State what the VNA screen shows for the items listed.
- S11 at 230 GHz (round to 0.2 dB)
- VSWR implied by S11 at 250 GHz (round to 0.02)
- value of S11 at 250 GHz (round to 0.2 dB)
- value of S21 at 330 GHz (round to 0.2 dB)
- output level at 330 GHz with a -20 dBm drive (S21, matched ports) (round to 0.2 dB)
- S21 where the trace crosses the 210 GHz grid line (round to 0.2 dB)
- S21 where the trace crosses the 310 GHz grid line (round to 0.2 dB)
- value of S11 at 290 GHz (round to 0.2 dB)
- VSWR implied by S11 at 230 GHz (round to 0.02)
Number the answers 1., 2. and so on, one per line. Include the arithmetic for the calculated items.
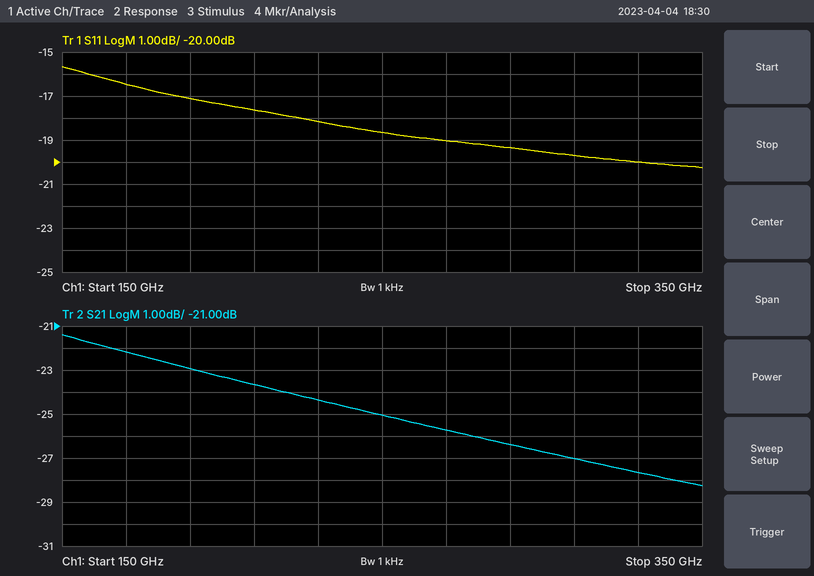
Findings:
1. -18.2 dB
2. |Γ| = 10^(-18.6/20) = 0.1175; VSWR = (1 + 0.1175)/(1 − 0.1175) ≈ 1.27, so 1.26 to the nearest 0.02
3. -18.6 dB
4. -27.6 dB
5. -20 dBm + (-27.6 dB) = -47.6 dBm
6. -23.6 dB
7. -27.0 dB
8. -19.4 dB
9. |Γ| = 10^(-18.2/20) = 0.1230; VSWR = (1 + 0.1230)/(1 − 0.1230) ≈ 1.28
